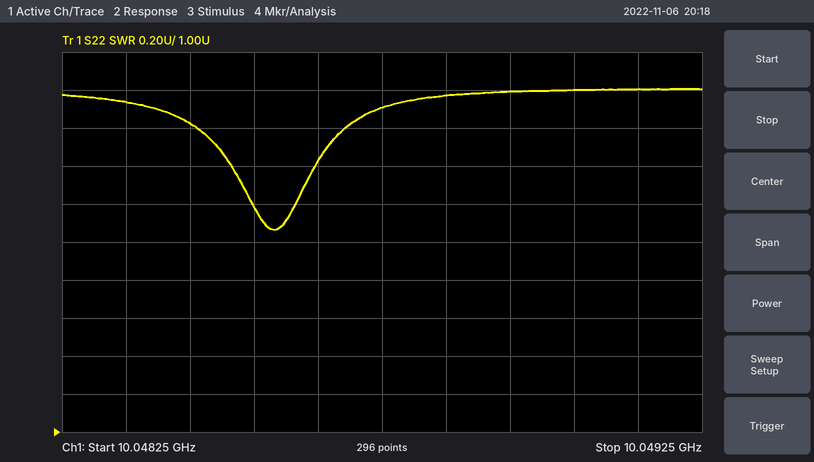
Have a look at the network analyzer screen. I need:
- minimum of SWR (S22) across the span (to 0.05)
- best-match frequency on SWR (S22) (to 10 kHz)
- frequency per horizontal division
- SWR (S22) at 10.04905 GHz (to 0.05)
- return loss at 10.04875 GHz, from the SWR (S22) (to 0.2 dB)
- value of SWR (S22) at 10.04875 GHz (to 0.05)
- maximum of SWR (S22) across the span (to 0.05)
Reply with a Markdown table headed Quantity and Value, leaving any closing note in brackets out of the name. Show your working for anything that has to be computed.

| Quantity | Value |
|---|---|
| minimum of SWR (S22) across the span | 2.05 |
| best-match frequency on SWR (S22) | 10.04858 GHz |
| frequency per horizontal division | 100 kHz |
| SWR (S22) at 10.04905 GHz | 2.80 |
| return loss at 10.04875 GHz, from the SWR (S22) | −20 log10((2.7 − 1)/(2.7 + 1)) ≈ 6.8 dB |
| value of SWR (S22) at 10.04875 GHz | 2.70 |
| maximum of SWR (S22) across the span | 2.80 |
